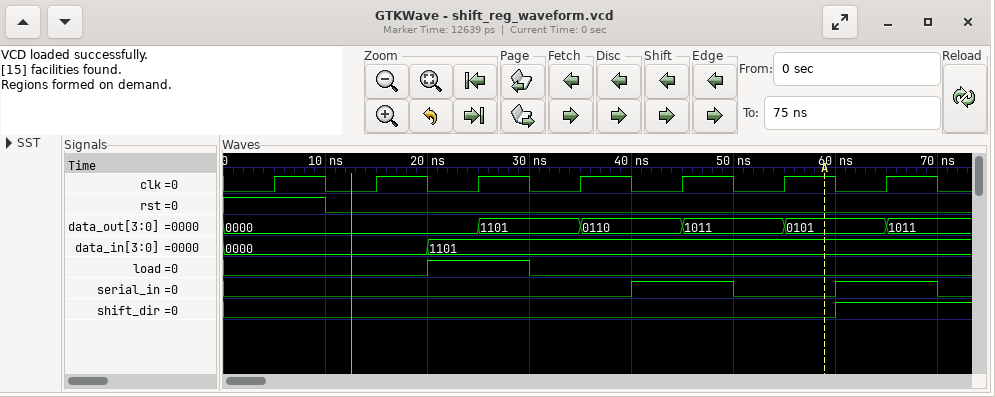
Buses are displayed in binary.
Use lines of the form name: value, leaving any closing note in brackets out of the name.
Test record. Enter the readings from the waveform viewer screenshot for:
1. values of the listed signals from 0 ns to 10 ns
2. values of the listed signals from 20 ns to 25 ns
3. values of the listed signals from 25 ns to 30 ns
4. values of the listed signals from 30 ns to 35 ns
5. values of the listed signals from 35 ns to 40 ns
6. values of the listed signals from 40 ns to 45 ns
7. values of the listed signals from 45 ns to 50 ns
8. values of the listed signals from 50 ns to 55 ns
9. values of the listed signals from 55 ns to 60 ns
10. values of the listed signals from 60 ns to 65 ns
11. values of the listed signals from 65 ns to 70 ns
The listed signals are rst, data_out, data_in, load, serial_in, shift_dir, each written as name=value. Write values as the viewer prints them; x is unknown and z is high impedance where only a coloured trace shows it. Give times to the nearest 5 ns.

values of the listed signals from 0 ns to 10 ns: rst=1, data_out=0000, data_in=0000, load=0, serial_in=0, shift_dir=0
values of the listed signals from 20 ns to 25 ns: rst=0, data_out=0000, data_in=1101, load=1, serial_in=0, shift_dir=0
values of the listed signals from 25 ns to 30 ns: rst=0, data_out=1101, data_in=1101, load=1, serial_in=0, shift_dir=0
values of the listed signals from 30 ns to 35 ns: rst=0, data_out=1101, data_in=1101, load=0, serial_in=0, shift_dir=0
values of the listed signals from 35 ns to 40 ns: rst=0, data_out=0110, data_in=1101, load=0, serial_in=0, shift_dir=0
values of the listed signals from 40 ns to 45 ns: rst=0, data_out=0110, data_in=1101, load=0, serial_in=1, shift_dir=0
values of the listed signals from 45 ns to 50 ns: rst=0, data_out=1011, data_in=1101, load=0, serial_in=1, shift_dir=0
values of the listed signals from 50 ns to 55 ns: rst=0, data_out=1011, data_in=1101, load=0, serial_in=0, shift_dir=0
values of the listed signals from 55 ns to 60 ns: rst=0, data_out=0101, data_in=1101, load=0, serial_in=0, shift_dir=0
values of the listed signals from 60 ns to 65 ns: rst=0, data_out=0101, data_in=1101, load=0, serial_in=1, shift_dir=1
values of the listed signals from 65 ns to 70 ns: rst=0, data_out=1011, data_in=1101, load=0, serial_in=1, shift_dir=1
